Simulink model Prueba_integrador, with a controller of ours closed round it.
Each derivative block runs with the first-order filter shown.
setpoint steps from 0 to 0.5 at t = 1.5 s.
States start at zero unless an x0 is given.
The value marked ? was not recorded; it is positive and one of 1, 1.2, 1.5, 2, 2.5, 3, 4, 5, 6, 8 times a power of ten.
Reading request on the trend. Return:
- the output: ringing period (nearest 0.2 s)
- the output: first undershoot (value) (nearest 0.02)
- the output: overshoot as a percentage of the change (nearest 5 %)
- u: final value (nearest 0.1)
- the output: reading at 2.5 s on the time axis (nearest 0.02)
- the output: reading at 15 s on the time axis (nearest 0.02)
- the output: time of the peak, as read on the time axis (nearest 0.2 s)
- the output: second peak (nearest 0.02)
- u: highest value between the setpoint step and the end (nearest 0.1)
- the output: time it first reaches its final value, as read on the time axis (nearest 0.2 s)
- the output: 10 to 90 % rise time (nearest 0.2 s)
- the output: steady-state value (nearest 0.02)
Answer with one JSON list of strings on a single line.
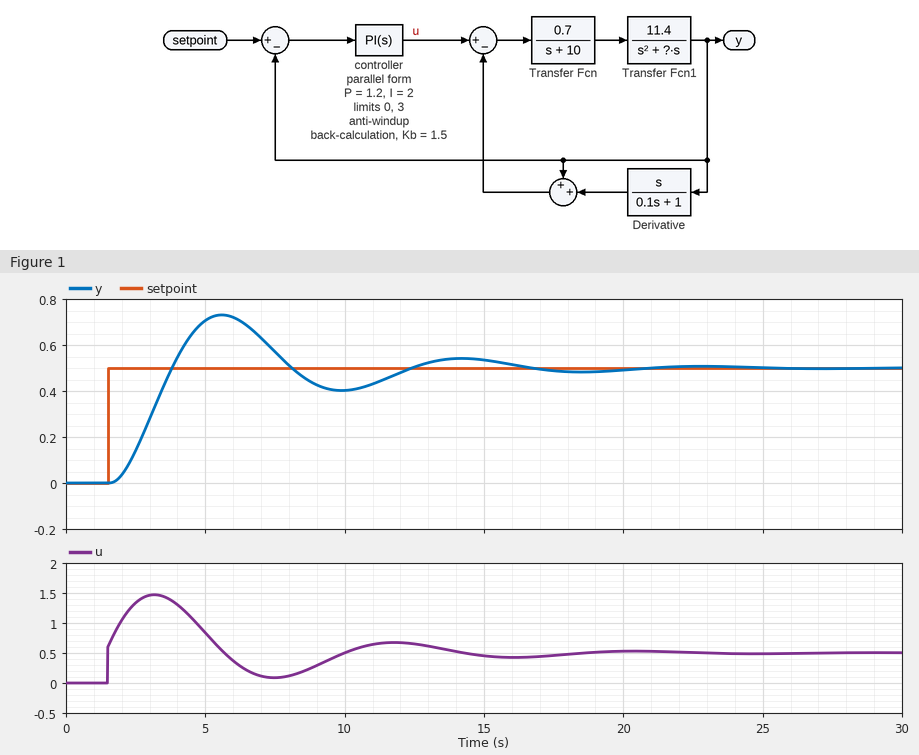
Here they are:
["8.6 s", "0.40", "45 %", "0.5", "0.14", "0.54", "5.6 s", "0.54", "1.5", "3.8 s", "1.6 s", "0.50"]
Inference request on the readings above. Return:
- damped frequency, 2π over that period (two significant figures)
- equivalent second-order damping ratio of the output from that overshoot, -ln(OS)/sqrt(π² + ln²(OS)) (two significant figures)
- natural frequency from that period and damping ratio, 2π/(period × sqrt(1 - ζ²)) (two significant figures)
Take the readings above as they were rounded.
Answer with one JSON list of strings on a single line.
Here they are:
["0.73 rad/s", "0.25", "0.75 rad/s"]
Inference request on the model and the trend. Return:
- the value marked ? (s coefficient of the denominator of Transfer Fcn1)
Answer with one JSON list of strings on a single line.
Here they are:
["2.5"]
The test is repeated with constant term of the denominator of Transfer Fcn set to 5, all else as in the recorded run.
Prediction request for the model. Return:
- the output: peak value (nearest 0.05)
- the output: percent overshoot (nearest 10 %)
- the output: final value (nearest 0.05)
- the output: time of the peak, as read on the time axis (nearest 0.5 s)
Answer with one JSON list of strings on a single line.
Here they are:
["0.70", "40 %", "0.50", "4.5 s"]
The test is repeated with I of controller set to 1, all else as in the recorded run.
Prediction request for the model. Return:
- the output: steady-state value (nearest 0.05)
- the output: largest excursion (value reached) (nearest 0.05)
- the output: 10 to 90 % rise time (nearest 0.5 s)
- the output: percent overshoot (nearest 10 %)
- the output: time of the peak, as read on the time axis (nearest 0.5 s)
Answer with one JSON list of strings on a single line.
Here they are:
["0.50", "0.60", "2.5 s", "20 %", "7.0 s"]
